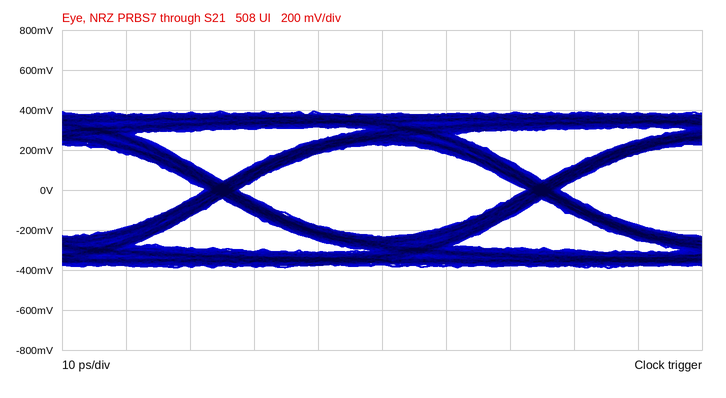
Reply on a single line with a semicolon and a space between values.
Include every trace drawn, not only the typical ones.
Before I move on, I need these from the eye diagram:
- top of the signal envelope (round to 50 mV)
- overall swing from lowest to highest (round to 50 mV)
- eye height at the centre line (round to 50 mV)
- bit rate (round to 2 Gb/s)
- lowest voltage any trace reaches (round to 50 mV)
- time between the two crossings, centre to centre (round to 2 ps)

400 mV; 800 mV; 450 mV; 20 Gb/s; -400 mV; 50 ps
